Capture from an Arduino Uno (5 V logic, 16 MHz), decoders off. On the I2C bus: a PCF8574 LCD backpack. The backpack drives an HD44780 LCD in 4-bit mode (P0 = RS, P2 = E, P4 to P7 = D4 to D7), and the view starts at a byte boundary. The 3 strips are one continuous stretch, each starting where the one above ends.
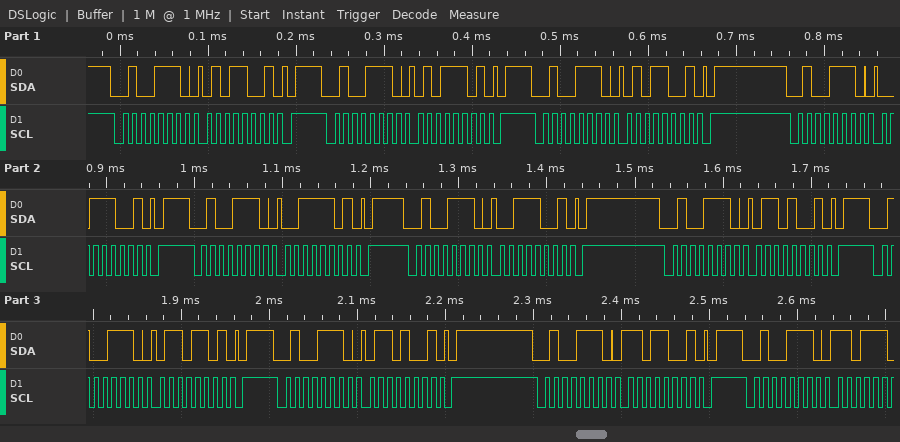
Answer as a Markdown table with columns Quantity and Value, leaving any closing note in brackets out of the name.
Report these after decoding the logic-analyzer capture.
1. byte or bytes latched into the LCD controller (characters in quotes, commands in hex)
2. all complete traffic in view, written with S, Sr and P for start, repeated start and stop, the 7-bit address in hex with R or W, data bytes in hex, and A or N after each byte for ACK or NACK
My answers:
| Quantity | Value |
|---|---|
| byte or bytes latched into the LCD controller | 'S' |
| all complete traffic in view, written with S, Sr and P for start, repeated start and stop, the 7-bit address in hex with R or W, data bytes in hex, and A or N after each byte for ACK or NACK | S 27W A 59 A P S 27W A 5D A P S 27W A 59 A P S 27W A 39 A P S 27W A 3D A P S 27W A 39 A P S 27W A 69 A P S 27W A 6D A P S 27W A 69 A P S 27W A D9 A P S 27W A |
